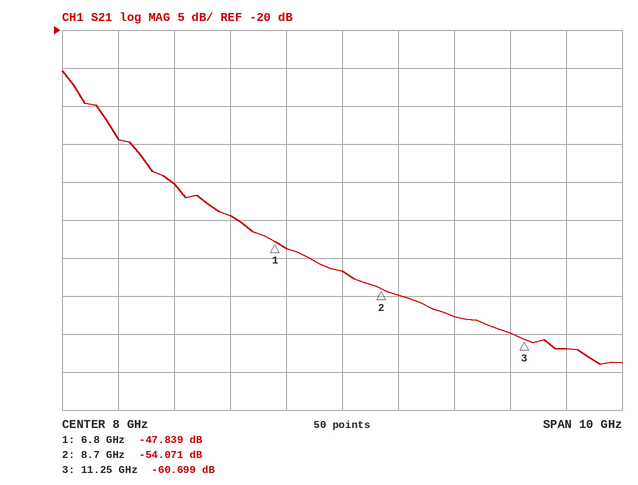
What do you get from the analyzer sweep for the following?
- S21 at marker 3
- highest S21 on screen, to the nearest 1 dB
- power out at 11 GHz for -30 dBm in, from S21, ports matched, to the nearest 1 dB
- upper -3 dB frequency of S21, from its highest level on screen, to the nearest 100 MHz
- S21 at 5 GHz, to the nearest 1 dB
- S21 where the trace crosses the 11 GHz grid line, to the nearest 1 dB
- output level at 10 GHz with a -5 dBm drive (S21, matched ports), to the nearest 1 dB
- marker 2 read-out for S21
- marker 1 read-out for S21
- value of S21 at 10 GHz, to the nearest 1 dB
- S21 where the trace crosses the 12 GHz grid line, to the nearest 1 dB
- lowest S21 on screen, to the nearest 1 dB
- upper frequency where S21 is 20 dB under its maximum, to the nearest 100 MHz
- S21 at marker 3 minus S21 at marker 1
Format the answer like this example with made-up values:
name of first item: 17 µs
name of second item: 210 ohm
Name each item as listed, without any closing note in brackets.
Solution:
S21 at marker 3: -60.699 dB
highest S21 on screen, to the nearest 1 dB: -25 dB
power out at 11 GHz for -30 dBm in, from S21, ports matched, to the nearest 1 dB: -90 dBm
upper -3 dB frequency of S21, from its highest level on screen, to the nearest 100 MHz: 3.3 GHz
S21 at 5 GHz, to the nearest 1 dB: -40 dB
S21 where the trace crosses the 11 GHz grid line, to the nearest 1 dB: -60 dB
output level at 10 GHz with a -5 dBm drive (S21, matched ports), to the nearest 1 dB: -63 dBm
marker 2 read-out for S21: -54.071 dB
marker 1 read-out for S21: -47.839 dB
value of S21 at 10 GHz, to the nearest 1 dB: -58 dB
S21 where the trace crosses the 12 GHz grid line, to the nearest 1 dB: -62 dB
lowest S21 on screen, to the nearest 1 dB: -64 dB
upper frequency where S21 is 20 dB under its maximum, to the nearest 100 MHz: 6.2 GHz
S21 at marker 3 minus S21 at marker 1: -12.860 dB
